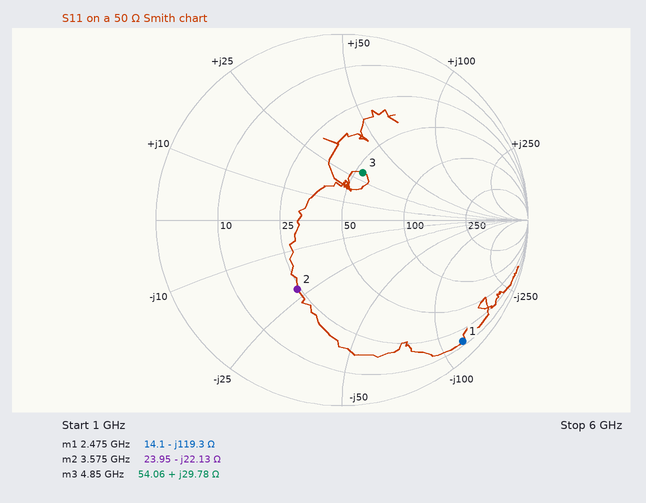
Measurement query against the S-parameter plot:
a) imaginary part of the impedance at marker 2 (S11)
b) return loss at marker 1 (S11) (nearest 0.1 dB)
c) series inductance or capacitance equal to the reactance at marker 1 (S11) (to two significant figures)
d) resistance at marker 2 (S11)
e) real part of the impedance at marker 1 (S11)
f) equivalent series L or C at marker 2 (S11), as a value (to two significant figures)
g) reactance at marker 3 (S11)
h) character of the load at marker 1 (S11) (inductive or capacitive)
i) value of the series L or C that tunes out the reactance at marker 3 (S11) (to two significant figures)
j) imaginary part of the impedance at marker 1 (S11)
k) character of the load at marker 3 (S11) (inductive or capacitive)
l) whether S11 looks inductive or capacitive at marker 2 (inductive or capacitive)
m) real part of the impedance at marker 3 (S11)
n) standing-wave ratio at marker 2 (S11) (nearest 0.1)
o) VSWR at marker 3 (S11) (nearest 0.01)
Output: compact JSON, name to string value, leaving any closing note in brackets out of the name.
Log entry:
{"imaginary part of the impedance at marker 2": "-22.13 Ω", "return loss at marker 1 (S11)": "0.7 dB", "series inductance or capacitance equal to the reactance at marker 1 (S11)": "540 fF", "resistance at marker 2": "23.95 Ω", "real part of the impedance at marker 1": "14.1 Ω", "equivalent series L or C at marker 2 (S11), as a value": "2.0 pF", "reactance at marker 3": "+29.78 Ω", "character of the load at marker 1 (S11)": "capacitive", "value of the series L or C that tunes out the reactance at marker 3 (S11)": "1.1 pF", "imaginary part of the impedance at marker 1": "-119.3 Ω", "character of the load at marker 3 (S11)": "inductive", "whether S11 looks inductive or capacitive at marker 2": "capacitive", "real part of the impedance at marker 3": "54.06 Ω", "standing-wave ratio at marker 2 (S11)": "2.6", "VSWR at marker 3 (S11)": "1.77"}
